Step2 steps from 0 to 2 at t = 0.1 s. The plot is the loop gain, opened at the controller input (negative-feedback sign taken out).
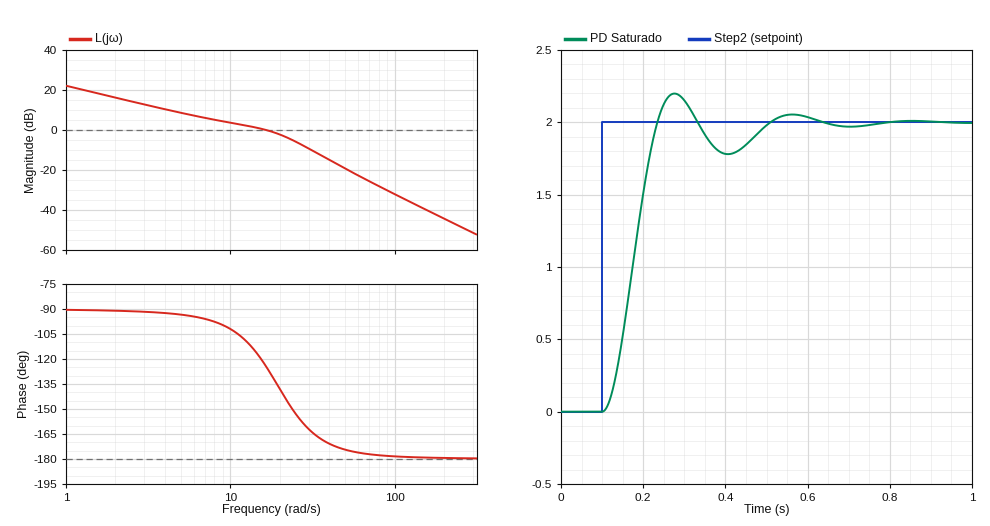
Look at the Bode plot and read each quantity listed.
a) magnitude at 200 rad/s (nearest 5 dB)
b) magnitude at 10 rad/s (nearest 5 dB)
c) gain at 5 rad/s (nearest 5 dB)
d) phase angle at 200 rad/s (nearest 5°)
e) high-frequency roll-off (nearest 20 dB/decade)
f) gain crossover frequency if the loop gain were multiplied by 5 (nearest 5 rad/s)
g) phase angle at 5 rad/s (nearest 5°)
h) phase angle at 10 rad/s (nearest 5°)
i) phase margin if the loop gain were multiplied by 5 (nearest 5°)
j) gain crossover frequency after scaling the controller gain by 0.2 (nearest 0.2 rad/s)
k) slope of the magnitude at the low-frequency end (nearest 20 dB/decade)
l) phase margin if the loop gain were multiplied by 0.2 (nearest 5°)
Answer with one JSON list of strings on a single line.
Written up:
["-45 dB", "5 dB", "10 dB", "-180°", "-40 dB/decade", "40 rad/s", "-95°", "-100°", "10°", "2.6 rad/s", "-20 dB/decade", "90°"]
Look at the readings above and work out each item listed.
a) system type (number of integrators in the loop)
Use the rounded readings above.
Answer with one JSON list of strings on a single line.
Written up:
["1"]
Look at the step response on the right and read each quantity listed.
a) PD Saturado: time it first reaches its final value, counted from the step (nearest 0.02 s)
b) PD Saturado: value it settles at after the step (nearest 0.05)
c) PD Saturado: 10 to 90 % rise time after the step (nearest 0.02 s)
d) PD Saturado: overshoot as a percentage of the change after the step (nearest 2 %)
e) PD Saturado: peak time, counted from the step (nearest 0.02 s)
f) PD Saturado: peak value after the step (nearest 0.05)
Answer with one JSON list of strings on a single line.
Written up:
["0.14 s", "2.00", "0.08 s", "10 %", "0.18 s", "2.20"]
